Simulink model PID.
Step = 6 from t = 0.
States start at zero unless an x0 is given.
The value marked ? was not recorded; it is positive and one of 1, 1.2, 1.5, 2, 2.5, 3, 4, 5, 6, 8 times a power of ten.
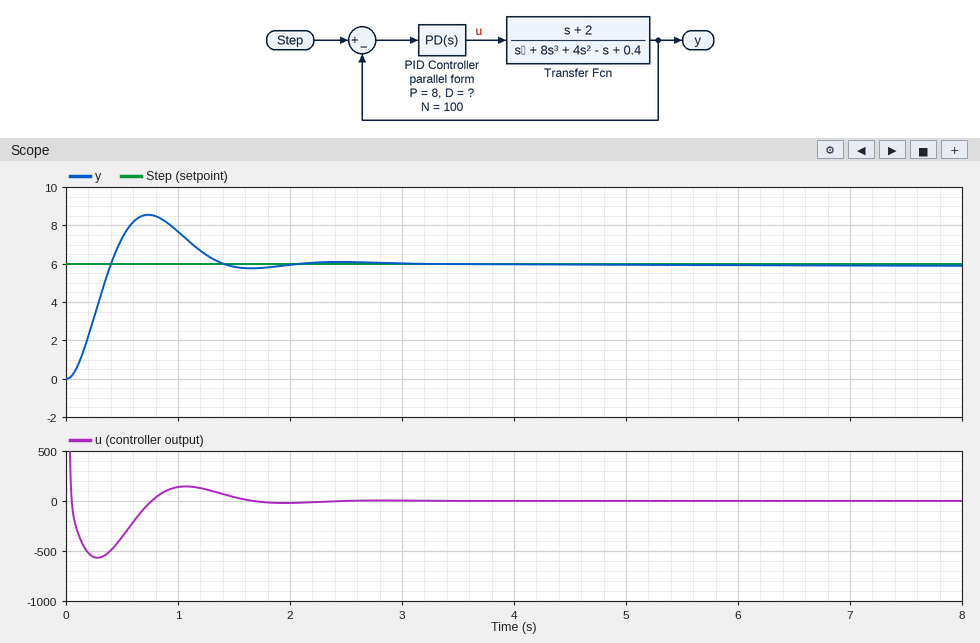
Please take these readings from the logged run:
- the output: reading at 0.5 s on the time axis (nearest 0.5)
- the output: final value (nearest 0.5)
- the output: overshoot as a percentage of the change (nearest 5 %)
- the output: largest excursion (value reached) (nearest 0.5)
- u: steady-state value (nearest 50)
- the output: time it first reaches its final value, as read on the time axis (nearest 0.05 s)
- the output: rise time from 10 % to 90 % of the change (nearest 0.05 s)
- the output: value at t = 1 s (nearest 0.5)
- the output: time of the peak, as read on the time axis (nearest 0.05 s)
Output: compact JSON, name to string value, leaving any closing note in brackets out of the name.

{"the output: reading at 0.5 s on the time axis": "7.5", "the output: final value": "6.0", "the output: overshoot as a percentage of the change": "45 %", "the output: largest excursion (value reached)": "8.5", "u: steady-state value": "0", "the output: time it first reaches its final value, as read on the time axis": "0.40 s", "the output: rise time from 10 % to 90 % of the change": "0.25 s", "the output: value at t = 1 s": "7.5", "the output: time of the peak, as read on the time axis": "0.75 s"}
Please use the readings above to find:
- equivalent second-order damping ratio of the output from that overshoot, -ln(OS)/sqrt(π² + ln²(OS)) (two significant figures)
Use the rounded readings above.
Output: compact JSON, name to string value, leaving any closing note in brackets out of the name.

{"equivalent second-order damping ratio of the output from that overshoot, -ln(OS)/sqrt(π² + ln²(OS))": "0.25"}
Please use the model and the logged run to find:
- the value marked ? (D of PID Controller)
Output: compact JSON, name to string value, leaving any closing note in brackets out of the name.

{"the value marked ?": "30"}
